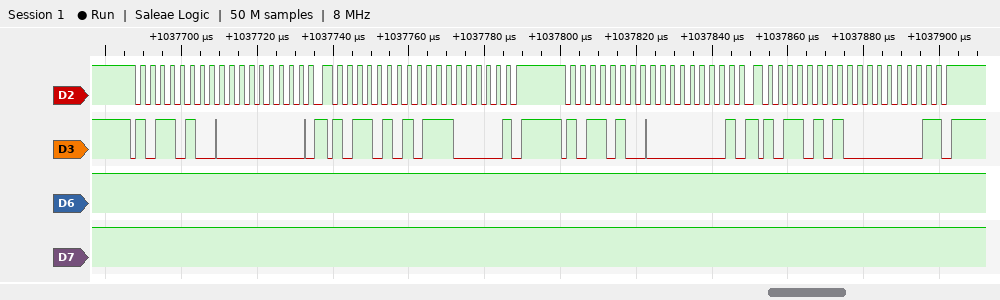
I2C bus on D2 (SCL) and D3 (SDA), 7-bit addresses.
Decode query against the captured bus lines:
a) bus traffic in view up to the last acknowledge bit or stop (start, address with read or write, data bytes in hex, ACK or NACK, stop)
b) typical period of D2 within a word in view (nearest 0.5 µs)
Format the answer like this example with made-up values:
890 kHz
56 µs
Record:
start, address 5A write ACK, 00 ACK, repeated start, address 5A read ACK, E0 NACK, stop, start, address 5A write ACK, 01 ACK, repeated start, address 5A read ACK, 01 NACK, stop
2.5 µs
